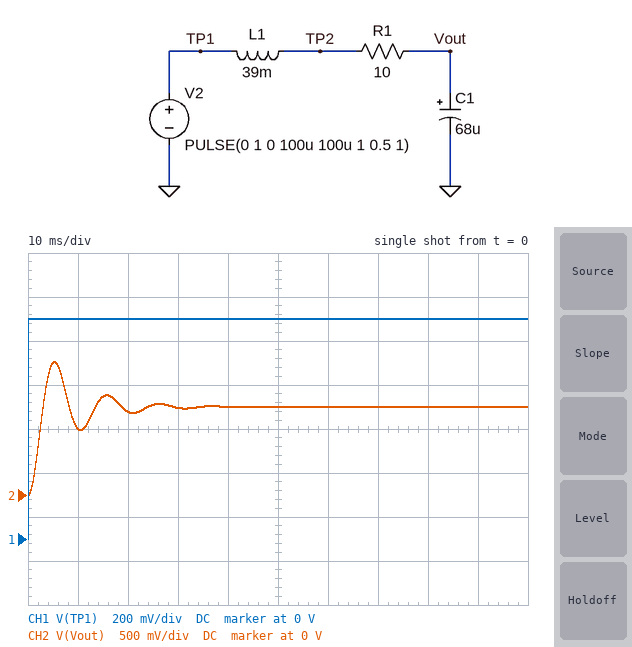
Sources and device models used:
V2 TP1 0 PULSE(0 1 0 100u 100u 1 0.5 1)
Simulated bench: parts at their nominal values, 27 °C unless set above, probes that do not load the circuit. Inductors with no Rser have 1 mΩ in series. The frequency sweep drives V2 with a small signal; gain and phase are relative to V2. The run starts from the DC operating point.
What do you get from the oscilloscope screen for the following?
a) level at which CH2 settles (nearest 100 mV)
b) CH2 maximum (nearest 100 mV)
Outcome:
1.0 V
1.5 V
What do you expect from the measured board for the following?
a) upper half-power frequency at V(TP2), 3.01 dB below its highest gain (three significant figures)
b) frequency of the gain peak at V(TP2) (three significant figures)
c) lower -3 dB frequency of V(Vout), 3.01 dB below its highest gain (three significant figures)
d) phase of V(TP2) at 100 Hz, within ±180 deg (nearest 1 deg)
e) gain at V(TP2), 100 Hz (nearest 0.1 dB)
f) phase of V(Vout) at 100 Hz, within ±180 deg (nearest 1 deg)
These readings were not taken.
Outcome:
113 Hz
94.0 Hz
69.4 Hz
-73 deg
8.1 dB
-96 deg
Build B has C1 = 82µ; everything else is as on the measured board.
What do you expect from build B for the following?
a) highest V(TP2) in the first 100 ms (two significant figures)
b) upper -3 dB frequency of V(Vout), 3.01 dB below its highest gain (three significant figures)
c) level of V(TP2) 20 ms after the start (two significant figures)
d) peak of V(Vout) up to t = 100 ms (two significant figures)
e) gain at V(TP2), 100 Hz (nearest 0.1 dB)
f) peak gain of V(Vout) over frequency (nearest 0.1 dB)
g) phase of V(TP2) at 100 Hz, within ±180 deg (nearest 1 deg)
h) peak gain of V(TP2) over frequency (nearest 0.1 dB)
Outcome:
1.5 V
103 Hz
990 mV
1.5 V
5.8 dB
7.0 dB
-90 deg
7.8 dB
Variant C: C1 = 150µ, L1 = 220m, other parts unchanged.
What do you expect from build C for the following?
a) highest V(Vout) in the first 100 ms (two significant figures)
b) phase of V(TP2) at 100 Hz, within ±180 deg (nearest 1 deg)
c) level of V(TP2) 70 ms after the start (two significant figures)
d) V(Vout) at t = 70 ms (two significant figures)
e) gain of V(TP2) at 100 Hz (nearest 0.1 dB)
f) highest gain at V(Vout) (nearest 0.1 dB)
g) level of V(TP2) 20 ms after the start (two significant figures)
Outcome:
1.7 V
-132 deg
810 mV
830 mV
-18.9 dB
11.7 dB
1.6 V
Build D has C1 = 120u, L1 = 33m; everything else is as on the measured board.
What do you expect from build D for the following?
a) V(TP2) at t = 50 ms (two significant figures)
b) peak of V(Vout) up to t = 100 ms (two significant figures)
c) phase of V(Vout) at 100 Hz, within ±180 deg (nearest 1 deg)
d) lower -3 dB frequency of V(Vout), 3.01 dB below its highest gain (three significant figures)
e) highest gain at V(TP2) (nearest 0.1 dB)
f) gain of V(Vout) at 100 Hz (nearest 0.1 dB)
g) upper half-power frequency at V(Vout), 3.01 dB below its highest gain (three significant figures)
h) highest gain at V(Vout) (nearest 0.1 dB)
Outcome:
1.0 V
1.4 V
-127 deg
39.4 Hz
6.0 dB
0.5 dB
94.4 Hz
4.8 dB
